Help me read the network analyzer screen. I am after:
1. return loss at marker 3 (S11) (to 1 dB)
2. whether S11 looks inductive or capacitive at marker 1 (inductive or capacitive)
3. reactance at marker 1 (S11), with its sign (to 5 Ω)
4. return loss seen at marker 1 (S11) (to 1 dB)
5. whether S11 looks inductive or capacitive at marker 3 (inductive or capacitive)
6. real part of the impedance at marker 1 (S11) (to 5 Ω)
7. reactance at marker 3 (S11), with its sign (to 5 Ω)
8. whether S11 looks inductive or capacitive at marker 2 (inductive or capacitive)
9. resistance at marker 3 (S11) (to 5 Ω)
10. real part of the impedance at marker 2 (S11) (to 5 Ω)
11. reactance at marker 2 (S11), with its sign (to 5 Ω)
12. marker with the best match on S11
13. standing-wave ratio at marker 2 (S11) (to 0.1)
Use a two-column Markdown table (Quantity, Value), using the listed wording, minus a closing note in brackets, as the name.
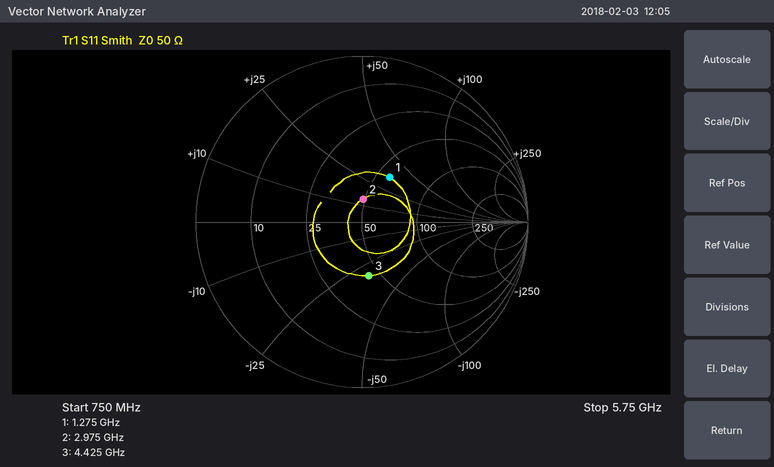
| Quantity | Value |
|---|---|
| return loss at marker 3 (S11) | 10 dB |
| whether S11 looks inductive or capacitive at marker 1 | inductive |
| reactance at marker 1 (S11), with its sign | +35 Ω |
| return loss seen at marker 1 (S11) | 10 dB |
| whether S11 looks inductive or capacitive at marker 3 | capacitive |
| real part of the impedance at marker 1 (S11) | 60 Ω |
| reactance at marker 3 (S11), with its sign | -30 Ω |
| whether S11 looks inductive or capacitive at marker 2 | inductive |
| resistance at marker 3 (S11) | 45 Ω |
| real part of the impedance at marker 2 (S11) | 50 Ω |
| reactance at marker 2 (S11), with its sign | +15 Ω |
| marker with the best match on S11 | marker 2 |
| standing-wave ratio at marker 2 (S11) | 1.3 |
